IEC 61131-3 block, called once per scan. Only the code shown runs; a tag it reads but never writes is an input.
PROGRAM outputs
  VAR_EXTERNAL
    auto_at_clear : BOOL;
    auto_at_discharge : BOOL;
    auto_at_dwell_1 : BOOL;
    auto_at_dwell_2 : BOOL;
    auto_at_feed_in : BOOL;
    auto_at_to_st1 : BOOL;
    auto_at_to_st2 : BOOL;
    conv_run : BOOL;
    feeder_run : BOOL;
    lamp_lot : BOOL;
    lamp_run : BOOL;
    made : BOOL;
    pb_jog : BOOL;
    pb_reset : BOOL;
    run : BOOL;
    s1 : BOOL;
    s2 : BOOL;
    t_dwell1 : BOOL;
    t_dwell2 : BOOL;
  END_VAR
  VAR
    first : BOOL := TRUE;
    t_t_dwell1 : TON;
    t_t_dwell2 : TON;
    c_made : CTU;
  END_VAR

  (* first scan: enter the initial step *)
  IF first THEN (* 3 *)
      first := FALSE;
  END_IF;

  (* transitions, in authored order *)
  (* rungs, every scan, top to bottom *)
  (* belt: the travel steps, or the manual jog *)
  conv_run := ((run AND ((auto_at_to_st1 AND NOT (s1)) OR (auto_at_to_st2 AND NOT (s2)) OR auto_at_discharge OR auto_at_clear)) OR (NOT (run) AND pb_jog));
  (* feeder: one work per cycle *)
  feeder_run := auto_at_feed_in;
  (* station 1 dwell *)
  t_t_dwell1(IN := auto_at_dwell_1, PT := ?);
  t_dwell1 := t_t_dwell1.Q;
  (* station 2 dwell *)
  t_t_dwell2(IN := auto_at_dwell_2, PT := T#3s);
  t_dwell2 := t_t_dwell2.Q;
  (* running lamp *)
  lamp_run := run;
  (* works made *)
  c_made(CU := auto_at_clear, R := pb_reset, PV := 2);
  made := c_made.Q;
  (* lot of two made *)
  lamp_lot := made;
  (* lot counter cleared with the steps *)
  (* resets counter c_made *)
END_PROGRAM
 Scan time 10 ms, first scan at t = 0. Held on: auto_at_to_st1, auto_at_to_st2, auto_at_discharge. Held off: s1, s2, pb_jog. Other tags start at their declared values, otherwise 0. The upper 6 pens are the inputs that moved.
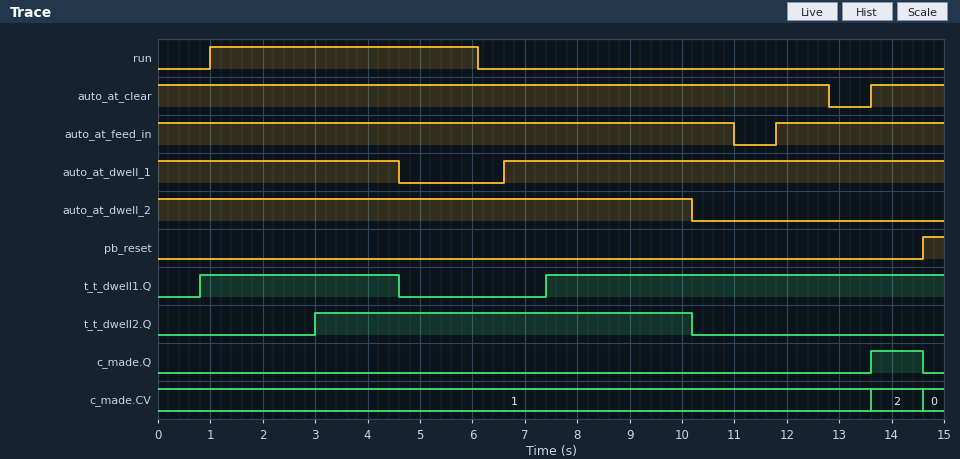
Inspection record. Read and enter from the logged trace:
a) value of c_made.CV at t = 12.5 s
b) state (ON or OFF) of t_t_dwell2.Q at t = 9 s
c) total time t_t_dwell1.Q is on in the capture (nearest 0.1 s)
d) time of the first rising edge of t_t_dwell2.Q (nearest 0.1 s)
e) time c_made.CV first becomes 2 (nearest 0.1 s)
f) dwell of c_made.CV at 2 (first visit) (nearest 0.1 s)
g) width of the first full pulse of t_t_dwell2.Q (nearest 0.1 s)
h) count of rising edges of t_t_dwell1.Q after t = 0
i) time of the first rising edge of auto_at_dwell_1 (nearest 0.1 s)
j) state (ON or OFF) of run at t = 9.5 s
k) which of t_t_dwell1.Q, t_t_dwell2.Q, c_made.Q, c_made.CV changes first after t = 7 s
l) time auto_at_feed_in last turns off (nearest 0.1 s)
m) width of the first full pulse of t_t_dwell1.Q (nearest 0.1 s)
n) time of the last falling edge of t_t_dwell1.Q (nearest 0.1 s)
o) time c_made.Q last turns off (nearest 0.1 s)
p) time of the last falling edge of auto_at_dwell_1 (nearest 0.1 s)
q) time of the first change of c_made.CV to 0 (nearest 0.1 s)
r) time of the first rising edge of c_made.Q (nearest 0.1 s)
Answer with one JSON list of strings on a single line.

["1", "ON", "11.4 s", "3.0 s", "13.6 s", "1.0 s", "7.2 s", "2", "6.6 s", "OFF", "t_t_dwell1.Q", "11.0 s", "3.8 s", "4.6 s", "14.6 s", "4.6 s", "14.6 s", "13.6 s"]
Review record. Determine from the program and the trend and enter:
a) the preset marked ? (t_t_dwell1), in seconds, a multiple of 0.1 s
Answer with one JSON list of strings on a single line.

["0.8 s"]
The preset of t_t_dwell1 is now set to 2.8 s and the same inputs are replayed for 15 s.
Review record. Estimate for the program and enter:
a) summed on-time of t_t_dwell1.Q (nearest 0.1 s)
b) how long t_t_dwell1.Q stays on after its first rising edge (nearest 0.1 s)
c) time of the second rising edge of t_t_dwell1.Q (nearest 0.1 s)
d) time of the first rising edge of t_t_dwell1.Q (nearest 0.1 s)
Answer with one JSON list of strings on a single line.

["7.4 s", "1.8 s", "9.4 s", "2.8 s"]
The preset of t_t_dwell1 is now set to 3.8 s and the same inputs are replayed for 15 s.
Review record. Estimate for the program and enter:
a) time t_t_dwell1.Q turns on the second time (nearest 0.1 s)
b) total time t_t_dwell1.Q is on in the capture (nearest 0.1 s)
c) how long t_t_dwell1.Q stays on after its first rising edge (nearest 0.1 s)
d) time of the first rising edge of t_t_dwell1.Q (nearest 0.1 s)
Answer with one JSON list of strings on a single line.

["10.4 s", "5.4 s", "0.8 s", "3.8 s"]
